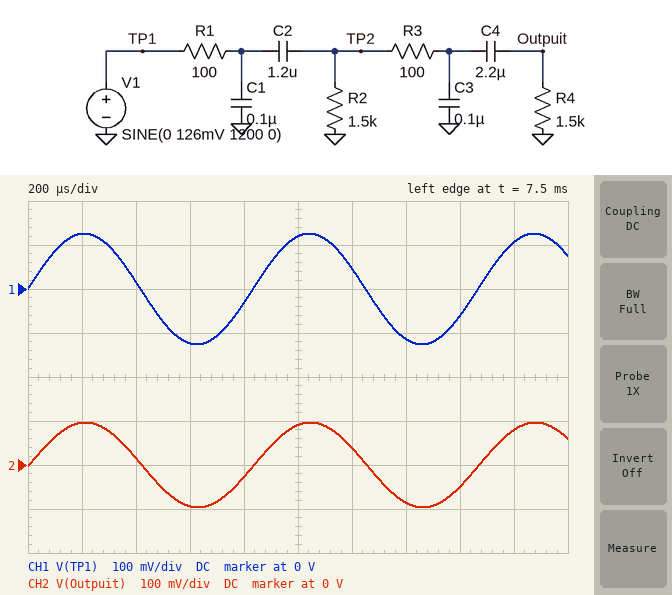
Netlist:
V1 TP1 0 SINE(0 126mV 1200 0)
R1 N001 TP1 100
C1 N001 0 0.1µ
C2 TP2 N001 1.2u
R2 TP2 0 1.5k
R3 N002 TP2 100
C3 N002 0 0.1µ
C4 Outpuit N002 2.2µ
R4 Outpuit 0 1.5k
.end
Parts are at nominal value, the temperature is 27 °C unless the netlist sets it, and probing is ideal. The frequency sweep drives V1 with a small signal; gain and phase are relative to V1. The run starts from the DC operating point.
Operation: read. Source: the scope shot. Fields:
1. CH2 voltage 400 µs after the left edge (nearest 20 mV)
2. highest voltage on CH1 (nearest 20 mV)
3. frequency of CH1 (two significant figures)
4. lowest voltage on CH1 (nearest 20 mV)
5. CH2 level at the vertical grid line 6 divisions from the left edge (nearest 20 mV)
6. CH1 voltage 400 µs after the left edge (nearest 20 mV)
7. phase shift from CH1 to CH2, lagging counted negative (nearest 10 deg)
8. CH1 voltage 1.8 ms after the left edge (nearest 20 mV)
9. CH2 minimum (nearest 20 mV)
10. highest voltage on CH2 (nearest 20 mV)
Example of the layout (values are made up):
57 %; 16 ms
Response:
20 mV; 120 mV; 1.2 kHz; -120 mV; 40 mV; 20 mV; 0 deg; 100 mV; -100 mV; 100 mV
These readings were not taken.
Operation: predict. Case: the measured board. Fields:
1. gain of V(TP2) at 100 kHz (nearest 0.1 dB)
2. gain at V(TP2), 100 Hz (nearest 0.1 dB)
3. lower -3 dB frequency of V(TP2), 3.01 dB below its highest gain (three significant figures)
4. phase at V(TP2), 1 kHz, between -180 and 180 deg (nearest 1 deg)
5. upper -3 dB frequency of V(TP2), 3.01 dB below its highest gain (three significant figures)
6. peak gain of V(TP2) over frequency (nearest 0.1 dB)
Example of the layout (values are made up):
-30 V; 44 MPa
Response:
-16.6 dB; -6.7 dB; 150 Hz; 2 deg; 9.32 kHz; -1.7 dB
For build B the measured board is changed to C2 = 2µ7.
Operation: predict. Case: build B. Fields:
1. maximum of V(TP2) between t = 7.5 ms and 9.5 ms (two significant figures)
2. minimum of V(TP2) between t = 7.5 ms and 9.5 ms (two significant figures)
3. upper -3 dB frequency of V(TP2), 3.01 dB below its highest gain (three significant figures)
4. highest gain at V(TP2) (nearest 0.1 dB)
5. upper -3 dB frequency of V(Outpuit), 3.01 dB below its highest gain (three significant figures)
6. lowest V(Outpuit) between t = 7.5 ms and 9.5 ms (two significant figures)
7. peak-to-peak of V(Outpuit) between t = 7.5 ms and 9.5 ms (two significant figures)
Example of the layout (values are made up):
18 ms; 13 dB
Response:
110 mV; -110 mV; 8.86 kHz; -1.4 dB; 7.24 kHz; -100 mV; 200 mV
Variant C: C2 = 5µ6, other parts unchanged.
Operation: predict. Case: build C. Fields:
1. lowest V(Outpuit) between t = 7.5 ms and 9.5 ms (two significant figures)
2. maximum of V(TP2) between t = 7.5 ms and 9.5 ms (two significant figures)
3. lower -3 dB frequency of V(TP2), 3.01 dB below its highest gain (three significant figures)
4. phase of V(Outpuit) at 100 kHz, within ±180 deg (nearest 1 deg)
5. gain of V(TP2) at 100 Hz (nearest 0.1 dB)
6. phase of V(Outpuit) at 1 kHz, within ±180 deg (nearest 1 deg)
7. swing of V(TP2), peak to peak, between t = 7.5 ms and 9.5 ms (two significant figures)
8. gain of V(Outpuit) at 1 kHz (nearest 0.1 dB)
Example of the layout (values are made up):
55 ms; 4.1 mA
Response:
-100 mV; 110 mV; 27.0 Hz; -153 deg; -1.9 dB; -5 deg; 220 mV; -1.8 dB
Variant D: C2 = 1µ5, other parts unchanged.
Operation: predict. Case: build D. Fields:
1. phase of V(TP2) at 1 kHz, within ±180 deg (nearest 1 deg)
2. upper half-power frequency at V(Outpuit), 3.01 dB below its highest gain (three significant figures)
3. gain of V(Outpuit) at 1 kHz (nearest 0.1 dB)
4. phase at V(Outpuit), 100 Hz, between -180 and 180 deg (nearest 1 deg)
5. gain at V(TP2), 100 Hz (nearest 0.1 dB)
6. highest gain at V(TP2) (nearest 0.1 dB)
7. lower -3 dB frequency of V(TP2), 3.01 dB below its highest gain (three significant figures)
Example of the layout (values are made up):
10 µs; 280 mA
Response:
1 deg; 7.41 kHz; -2.2 dB; 64 deg; -5.5 dB; -1.6 dB; 123 Hz
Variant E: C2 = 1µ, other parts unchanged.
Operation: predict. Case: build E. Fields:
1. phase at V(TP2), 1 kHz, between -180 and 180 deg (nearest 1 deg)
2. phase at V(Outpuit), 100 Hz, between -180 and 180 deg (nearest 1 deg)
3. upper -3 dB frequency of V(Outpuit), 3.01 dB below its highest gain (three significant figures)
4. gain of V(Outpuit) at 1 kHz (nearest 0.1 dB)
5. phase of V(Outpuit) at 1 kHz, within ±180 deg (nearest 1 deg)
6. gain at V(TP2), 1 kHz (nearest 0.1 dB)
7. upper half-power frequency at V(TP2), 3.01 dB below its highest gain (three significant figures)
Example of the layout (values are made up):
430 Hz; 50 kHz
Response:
4 deg; 73 deg; 7.60 kHz; -2.5 dB; 3 deg; -1.9 dB; 9.48 kHz
